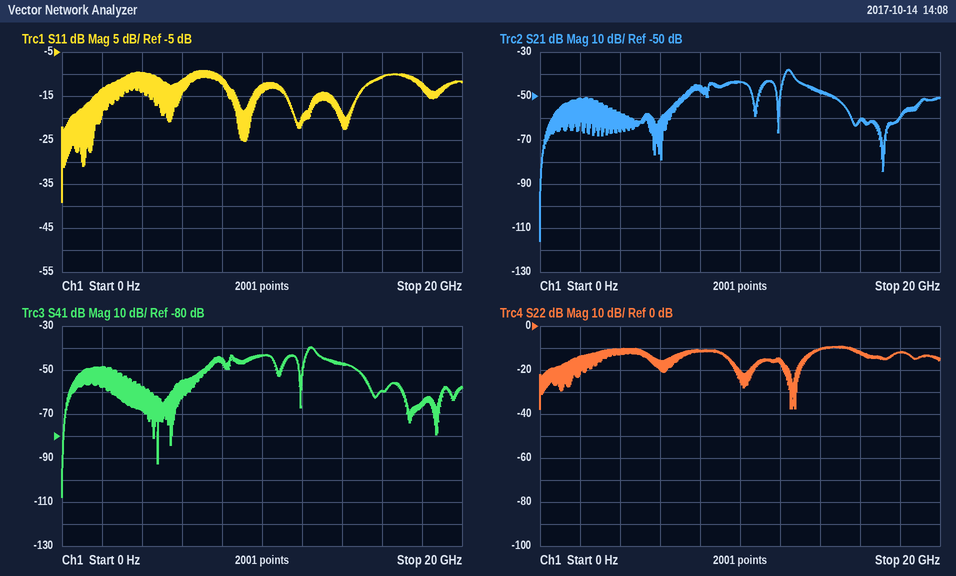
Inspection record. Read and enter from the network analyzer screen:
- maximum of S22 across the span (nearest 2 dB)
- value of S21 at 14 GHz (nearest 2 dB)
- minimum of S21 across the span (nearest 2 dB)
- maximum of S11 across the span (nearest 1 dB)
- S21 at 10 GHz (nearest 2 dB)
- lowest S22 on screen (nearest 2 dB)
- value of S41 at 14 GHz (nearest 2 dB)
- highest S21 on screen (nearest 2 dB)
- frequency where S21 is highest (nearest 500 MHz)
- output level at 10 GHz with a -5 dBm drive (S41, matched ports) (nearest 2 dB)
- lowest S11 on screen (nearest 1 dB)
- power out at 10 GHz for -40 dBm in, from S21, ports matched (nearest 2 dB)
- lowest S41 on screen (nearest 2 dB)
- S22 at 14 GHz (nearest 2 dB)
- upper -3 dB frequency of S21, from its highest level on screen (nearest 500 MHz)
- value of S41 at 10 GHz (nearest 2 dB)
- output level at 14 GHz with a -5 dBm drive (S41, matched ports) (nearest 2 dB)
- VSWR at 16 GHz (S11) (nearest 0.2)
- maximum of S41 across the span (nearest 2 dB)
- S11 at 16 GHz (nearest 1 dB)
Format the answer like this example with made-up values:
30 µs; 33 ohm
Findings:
-10 dB; -48 dB; -116 dB; -9 dB; -44 dB; -38 dB; -48 dB; -38 dB; 12.5 GHz; -48 dBm; -39 dB; -84 dBm; -108 dB; -10 dB; 12.5 GHz; -44 dB; -52 dBm; 1.8; -40 dB; -11 dB
